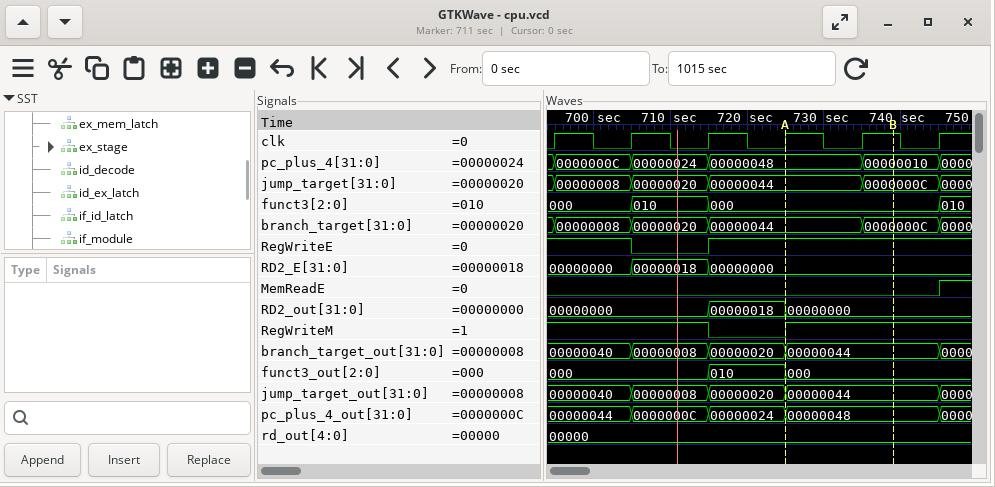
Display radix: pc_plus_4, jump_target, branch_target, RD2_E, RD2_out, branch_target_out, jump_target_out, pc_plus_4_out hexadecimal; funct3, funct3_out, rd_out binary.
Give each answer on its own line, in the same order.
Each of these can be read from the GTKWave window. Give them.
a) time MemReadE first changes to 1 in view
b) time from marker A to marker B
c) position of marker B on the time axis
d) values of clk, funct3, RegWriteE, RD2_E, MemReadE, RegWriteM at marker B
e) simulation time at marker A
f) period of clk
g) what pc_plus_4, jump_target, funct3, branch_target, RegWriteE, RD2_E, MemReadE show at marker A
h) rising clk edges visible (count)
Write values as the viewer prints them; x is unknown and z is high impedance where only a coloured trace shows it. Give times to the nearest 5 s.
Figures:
745 s
15 s
740 s
clk=1, funct3=000, RegWriteE=1, RD2_E=00000000, MemReadE=0, RegWriteM=1
725 s
10 s
pc_plus_4=00000048, jump_target=00000044, funct3=000, branch_target=00000044, RegWriteE=1, RD2_E=00000000, MemReadE=0
6
